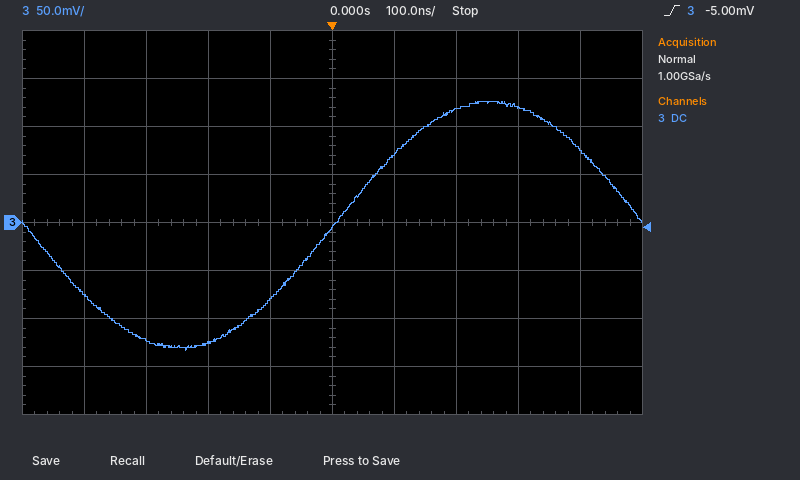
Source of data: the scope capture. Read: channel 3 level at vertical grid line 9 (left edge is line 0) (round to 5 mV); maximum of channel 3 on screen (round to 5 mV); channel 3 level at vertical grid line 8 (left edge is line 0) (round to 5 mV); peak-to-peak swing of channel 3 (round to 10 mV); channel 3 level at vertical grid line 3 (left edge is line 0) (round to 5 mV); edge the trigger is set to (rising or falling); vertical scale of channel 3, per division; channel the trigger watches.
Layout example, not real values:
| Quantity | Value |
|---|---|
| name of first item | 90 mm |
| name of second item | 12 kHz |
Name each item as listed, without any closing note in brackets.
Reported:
| Quantity | Value |
|---|---|
| channel 3 level at vertical grid line 9 (left edge is line 0) | 75 mV |
| maximum of channel 3 on screen | 125 mV |
| channel 3 level at vertical grid line 8 (left edge is line 0) | 120 mV |
| peak-to-peak swing of channel 3 | 260 mV |
| channel 3 level at vertical grid line 3 (left edge is line 0) | -125 mV |
| edge the trigger is set to | rising |
| vertical scale of channel 3, per division | 50 mV |
| channel the trigger watches | channel 3 |
